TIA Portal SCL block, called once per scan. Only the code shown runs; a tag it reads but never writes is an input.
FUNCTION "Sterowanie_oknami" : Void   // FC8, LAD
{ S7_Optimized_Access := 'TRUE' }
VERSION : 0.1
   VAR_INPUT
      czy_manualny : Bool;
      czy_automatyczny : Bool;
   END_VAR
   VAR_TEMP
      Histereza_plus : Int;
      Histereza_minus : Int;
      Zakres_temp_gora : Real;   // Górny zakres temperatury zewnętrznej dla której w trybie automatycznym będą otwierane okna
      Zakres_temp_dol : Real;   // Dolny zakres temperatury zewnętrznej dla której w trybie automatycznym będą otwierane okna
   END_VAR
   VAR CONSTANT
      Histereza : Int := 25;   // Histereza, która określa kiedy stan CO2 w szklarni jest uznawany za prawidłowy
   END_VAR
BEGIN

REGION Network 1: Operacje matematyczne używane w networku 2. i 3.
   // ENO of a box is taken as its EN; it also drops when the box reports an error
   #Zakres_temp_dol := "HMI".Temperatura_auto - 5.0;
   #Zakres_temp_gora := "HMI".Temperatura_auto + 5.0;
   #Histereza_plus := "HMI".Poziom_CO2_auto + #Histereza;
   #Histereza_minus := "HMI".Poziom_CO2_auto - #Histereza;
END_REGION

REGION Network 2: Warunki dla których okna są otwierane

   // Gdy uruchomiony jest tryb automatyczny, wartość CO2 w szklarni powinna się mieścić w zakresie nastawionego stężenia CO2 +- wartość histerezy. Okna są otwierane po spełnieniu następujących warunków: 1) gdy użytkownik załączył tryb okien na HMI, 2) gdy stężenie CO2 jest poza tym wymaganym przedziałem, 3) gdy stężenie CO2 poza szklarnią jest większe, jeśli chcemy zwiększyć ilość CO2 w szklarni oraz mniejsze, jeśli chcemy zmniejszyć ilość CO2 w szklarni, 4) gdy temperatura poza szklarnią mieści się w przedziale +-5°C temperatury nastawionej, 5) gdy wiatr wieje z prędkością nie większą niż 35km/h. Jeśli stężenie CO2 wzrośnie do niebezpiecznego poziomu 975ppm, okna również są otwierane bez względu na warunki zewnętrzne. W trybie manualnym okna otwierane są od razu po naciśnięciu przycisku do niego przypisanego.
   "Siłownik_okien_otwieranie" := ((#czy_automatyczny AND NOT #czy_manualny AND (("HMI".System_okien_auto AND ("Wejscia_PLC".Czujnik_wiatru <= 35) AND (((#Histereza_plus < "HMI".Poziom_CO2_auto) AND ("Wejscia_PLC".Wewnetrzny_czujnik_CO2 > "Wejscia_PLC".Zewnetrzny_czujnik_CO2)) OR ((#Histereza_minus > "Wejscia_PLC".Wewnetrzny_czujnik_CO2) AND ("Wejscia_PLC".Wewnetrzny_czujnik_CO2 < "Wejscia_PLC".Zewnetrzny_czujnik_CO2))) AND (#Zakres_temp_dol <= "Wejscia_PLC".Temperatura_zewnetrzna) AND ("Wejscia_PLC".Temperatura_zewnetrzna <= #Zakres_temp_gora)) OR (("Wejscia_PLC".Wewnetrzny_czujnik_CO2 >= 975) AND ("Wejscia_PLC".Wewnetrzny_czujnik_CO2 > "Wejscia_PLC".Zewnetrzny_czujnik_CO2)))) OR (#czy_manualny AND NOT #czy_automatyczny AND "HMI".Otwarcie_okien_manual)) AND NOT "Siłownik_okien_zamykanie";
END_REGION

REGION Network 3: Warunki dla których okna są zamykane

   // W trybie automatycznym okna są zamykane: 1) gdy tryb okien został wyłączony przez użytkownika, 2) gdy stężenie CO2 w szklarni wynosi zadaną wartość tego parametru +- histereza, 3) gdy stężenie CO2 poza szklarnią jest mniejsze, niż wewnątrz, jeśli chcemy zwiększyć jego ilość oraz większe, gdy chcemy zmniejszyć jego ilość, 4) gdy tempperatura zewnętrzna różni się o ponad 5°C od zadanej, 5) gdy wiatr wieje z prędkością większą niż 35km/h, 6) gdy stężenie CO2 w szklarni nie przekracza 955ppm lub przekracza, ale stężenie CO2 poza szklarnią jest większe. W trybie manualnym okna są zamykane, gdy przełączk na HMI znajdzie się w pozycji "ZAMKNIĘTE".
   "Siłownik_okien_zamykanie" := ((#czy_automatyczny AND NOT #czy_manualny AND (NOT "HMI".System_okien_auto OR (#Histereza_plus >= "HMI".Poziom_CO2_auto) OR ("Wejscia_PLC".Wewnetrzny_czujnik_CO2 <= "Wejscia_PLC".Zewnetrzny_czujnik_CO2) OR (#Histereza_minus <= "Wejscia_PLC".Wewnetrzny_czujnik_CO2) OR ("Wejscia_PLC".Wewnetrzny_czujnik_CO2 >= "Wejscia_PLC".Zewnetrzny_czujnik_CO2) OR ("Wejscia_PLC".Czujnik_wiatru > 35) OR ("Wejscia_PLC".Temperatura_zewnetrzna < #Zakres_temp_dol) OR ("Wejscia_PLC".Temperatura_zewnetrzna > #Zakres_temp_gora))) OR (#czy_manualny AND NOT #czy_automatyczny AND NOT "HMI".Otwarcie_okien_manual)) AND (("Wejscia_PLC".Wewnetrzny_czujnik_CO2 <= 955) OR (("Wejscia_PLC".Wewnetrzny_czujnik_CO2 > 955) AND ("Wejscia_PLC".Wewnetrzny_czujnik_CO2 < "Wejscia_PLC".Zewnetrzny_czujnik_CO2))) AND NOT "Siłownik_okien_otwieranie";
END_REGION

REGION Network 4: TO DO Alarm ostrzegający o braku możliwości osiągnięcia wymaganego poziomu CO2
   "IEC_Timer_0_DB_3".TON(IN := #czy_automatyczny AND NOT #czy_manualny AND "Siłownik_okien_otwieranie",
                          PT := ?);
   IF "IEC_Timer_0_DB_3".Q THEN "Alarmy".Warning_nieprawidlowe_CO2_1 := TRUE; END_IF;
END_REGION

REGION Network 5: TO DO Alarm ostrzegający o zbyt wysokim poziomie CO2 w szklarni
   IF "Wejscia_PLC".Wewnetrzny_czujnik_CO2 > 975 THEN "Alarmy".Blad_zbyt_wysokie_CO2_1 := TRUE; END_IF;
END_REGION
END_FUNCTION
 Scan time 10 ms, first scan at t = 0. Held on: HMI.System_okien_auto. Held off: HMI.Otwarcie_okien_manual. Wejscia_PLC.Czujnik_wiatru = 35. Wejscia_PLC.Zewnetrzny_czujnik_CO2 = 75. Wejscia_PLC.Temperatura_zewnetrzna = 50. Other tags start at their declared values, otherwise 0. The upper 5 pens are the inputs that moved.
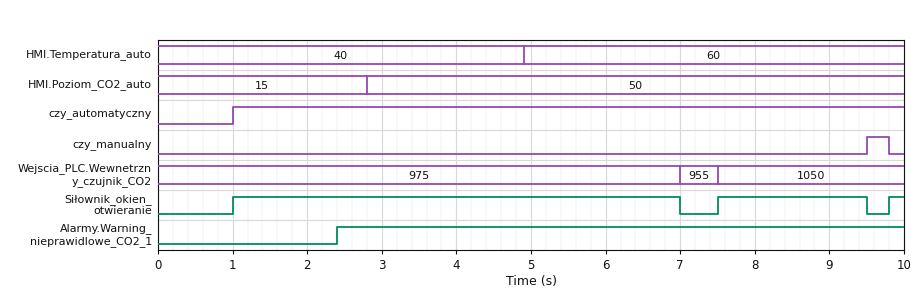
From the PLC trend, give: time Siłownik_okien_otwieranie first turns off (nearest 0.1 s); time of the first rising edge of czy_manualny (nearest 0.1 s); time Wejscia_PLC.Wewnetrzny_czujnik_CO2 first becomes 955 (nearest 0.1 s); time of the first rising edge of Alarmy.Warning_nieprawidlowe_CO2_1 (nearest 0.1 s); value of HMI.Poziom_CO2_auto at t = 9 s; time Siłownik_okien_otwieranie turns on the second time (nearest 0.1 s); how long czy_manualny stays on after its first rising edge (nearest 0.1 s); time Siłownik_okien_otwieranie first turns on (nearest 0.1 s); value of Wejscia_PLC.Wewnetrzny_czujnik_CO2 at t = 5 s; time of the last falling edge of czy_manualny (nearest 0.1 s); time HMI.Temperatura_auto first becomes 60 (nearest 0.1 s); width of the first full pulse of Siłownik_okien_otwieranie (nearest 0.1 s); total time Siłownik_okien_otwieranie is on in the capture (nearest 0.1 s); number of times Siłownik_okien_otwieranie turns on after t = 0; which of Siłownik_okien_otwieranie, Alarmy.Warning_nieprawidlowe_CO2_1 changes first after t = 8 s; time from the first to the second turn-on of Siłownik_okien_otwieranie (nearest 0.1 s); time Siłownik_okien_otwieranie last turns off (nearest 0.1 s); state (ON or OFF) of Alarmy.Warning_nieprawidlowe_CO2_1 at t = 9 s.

7.0 s
9.5 s
7.0 s
2.4 s
50
7.5 s
0.3 s
1.0 s
975
9.8 s
4.9 s
6.0 s
8.2 s
3
Siłownik_okien_otwieranie
6.5 s
9.5 s
ON
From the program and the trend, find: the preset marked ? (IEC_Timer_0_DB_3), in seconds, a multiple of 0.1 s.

1.4 s
